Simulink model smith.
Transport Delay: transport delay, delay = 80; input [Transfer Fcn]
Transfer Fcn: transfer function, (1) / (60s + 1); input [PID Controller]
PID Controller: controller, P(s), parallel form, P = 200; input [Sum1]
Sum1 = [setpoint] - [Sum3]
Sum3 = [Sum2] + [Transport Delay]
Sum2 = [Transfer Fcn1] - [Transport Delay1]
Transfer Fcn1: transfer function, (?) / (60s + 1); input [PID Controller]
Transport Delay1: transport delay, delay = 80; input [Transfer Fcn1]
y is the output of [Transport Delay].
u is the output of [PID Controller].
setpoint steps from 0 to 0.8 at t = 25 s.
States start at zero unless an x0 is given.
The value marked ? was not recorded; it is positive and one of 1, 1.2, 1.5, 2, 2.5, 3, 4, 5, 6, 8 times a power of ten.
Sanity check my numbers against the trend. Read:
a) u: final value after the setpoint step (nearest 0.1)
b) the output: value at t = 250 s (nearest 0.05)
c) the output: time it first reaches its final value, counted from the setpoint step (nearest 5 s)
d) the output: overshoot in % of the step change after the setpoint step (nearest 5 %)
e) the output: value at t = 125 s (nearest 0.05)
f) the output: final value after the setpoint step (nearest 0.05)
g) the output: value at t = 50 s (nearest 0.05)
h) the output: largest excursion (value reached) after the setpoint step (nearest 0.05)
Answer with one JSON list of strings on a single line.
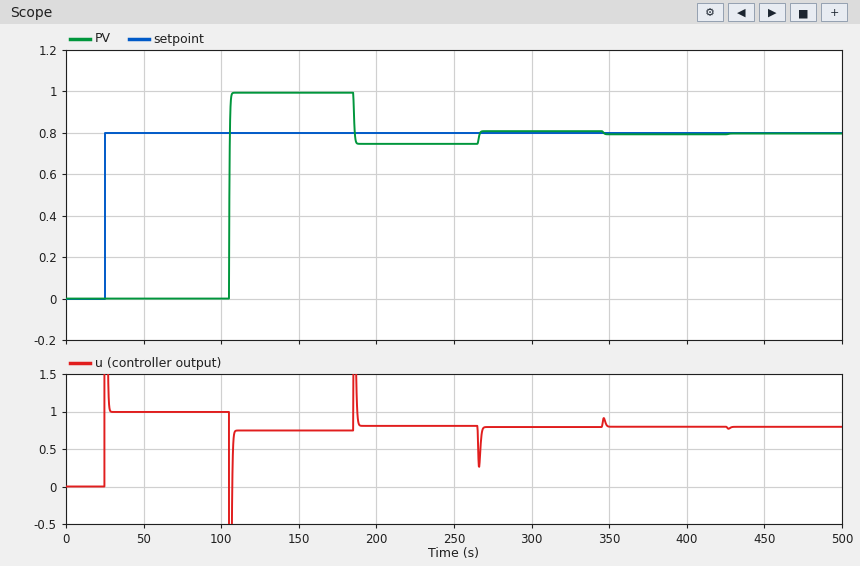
["0.8", "0.75", "80 s", "25 %", "1.00", "0.80", "0.00", "1.00"]
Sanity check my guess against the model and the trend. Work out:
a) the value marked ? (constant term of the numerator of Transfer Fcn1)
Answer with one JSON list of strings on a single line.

["0.8"]
